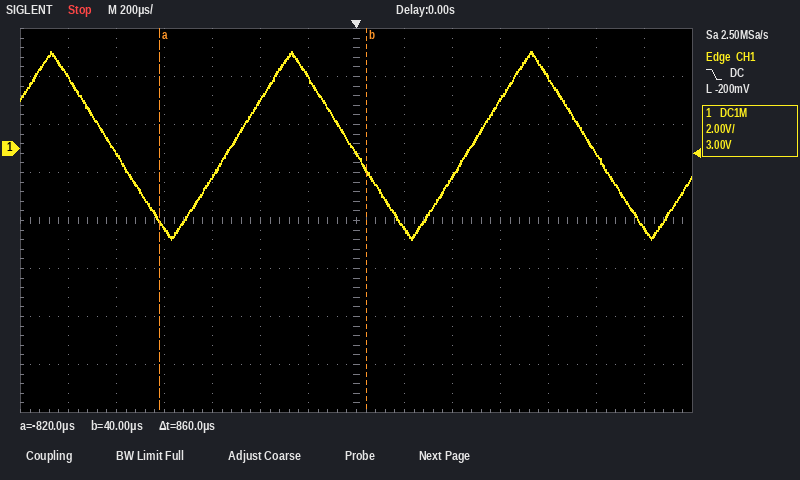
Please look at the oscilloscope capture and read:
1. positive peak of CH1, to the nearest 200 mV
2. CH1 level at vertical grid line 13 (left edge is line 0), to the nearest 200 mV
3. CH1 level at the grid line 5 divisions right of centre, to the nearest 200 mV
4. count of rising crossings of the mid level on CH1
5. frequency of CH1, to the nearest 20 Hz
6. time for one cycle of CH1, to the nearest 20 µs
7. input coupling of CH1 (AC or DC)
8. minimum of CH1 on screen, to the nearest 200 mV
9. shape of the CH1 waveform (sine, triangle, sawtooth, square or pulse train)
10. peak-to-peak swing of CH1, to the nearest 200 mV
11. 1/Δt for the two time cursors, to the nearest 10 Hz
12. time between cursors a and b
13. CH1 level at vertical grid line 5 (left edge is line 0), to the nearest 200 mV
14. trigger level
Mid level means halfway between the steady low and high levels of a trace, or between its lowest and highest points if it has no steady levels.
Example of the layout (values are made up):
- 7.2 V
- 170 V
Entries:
- 4.0 V
- -3.4 V
- -200 mV
- 2
- 1.00 kHz
- 1.00 ms
- DC
- -3.8 V
- triangle
- 7.8 V
- 1.16 kHz
- 860 µs
- 2.0 V
- -200 mV
